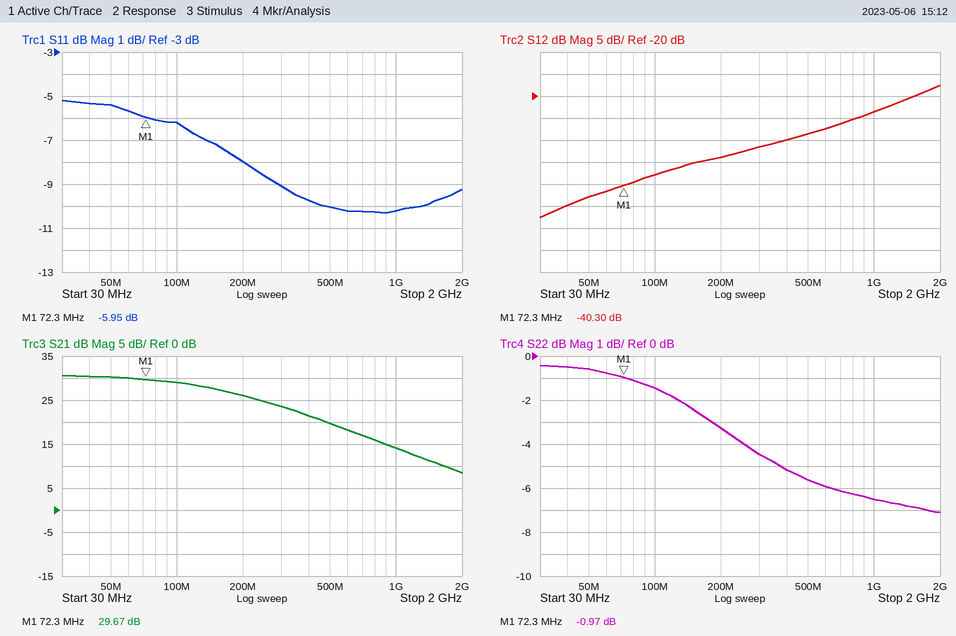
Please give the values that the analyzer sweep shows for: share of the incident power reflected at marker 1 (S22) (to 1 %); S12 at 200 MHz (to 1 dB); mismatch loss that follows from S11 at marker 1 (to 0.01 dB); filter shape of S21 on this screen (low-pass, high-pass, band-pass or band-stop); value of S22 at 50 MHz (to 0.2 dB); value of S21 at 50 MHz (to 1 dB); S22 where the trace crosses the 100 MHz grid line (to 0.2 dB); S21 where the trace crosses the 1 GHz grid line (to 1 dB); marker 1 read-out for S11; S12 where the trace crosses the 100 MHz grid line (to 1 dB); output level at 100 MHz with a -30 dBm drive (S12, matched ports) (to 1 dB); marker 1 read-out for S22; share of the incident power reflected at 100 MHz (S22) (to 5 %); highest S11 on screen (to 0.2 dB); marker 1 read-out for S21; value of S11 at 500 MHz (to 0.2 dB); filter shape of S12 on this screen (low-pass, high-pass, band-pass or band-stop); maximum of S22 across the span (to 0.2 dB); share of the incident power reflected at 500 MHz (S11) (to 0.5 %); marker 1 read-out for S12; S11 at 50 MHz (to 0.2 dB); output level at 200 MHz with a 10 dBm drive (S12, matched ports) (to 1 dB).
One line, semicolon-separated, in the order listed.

80 %; -34 dB; 1.27 dB; low-pass; -0.6 dB; 30 dB; -1.4 dB; 14 dB; -5.95 dB; -38 dB; -68 dBm; -0.97 dB; 70 %; -5.2 dB; 29.67 dB; -10.0 dB; high-pass; -0.4 dB; 10.0 %; -40.30 dB; -5.4 dB; -24 dBm
